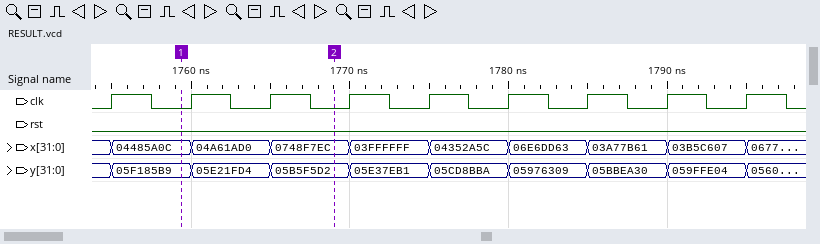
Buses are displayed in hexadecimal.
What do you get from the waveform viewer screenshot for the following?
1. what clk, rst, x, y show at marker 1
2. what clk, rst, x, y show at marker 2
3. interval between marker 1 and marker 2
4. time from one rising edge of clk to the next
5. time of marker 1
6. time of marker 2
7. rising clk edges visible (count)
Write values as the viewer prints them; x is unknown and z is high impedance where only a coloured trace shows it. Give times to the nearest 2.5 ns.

clk=0, rst=0, x=04485A0C, y=05F185B9
clk=0, rst=0, x=0748F7EC, y=05B5F5D2
10 ns
5 ns
1760 ns
1770 ns
9
